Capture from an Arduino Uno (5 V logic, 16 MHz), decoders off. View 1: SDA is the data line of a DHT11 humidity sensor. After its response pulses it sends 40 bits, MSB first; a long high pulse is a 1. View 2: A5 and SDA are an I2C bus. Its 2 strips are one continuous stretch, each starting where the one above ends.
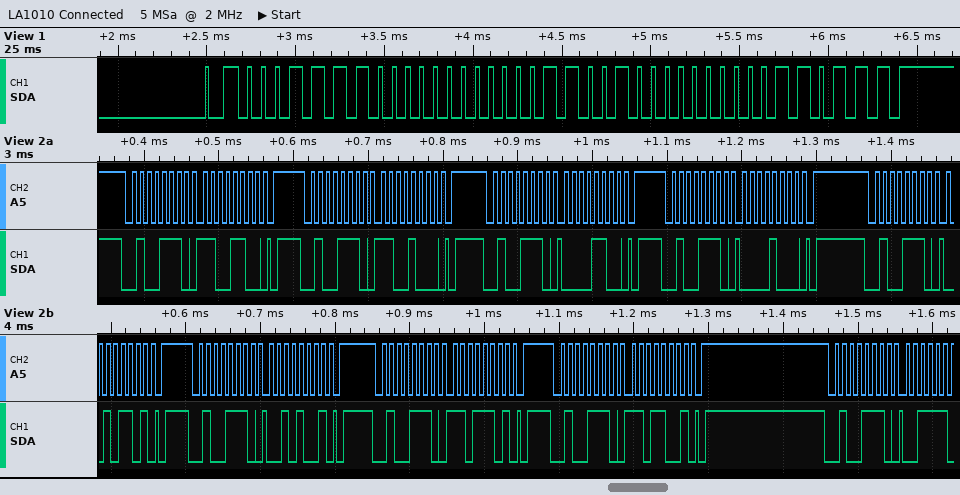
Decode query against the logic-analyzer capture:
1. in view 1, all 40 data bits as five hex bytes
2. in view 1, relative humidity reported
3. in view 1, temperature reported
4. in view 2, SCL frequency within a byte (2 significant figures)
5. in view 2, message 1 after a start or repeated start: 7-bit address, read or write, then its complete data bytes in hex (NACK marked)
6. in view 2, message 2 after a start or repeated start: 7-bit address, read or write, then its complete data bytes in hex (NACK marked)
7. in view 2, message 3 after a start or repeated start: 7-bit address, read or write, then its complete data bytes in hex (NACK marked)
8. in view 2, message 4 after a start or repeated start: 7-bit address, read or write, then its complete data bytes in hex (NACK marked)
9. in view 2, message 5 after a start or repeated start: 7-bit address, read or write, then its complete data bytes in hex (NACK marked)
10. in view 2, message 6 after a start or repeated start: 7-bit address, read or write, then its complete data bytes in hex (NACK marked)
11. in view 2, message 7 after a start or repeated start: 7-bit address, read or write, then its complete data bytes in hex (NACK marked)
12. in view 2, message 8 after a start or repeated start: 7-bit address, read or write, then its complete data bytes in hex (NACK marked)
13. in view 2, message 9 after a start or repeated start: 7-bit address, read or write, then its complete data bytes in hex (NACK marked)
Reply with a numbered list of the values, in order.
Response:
1. 1E 00 19 00 37
2. 30 %
3. 25.0 °C
4. 100 kHz
5. 0x27 write: CC
6. 0x27 write: C8
7. 0x27 write: 0C
8. 0x27 write: 08
9. 0x27 write: 2D
10. 0x27 write: 29
11. 0x27 write: DD
12. 0x27 write: D9
13. 0x27 write
